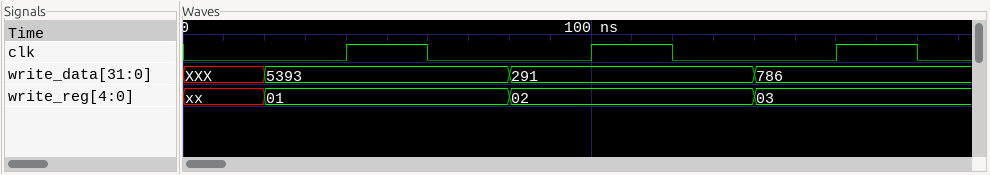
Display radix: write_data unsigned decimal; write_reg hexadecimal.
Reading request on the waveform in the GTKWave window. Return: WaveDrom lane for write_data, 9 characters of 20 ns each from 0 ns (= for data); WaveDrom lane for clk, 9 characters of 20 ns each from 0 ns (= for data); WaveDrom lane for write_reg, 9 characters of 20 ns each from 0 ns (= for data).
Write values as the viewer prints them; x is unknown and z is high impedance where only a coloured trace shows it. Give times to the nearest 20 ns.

{name: 'write_data', wave: 'x=..=..=.', data: '5393 291 786'}
{name: 'clk', wave: '0.10.10.1'}
{name: 'write_reg', wave: 'x=..=..=.', data: '01 02 03'}
